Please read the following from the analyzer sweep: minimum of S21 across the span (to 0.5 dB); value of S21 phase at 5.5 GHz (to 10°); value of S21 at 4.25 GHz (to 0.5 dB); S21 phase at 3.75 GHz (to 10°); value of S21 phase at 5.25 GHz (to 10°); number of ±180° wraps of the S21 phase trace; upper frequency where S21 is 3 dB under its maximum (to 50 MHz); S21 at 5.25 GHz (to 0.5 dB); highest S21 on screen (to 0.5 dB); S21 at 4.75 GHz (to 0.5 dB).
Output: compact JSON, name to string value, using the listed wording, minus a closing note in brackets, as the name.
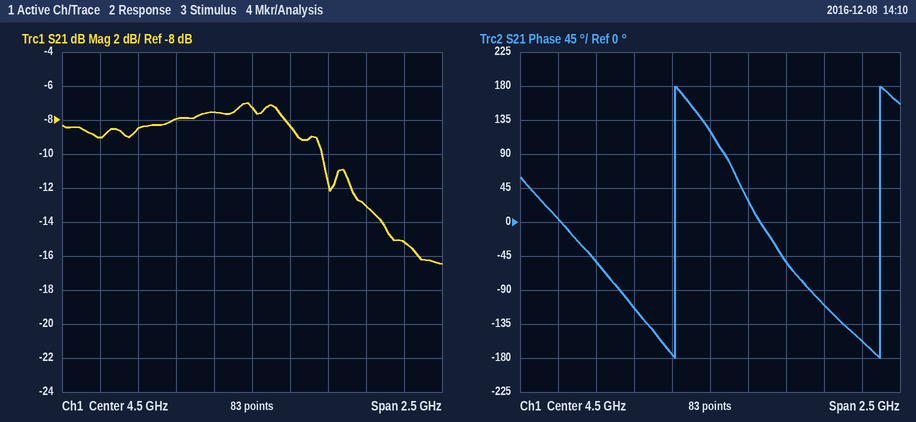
{"minimum of S21 across the span": "-16.5 dB", "value of S21 phase at 5.5 GHz": "-160°", "value of S21 at 4.25 GHz": "-7.5 dB", "S21 phase at 3.75 GHz": "-50°", "value of S21 phase at 5.25 GHz": "-110°", "number of ±180° wraps of the S21 phase trace": "2", "upper frequency where S21 is 3 dB under its maximum": "4.95 GHz", "S21 at 5.25 GHz": "-13.0 dB", "highest S21 on screen": "-7.0 dB", "S21 at 4.75 GHz": "-8.5 dB"}
